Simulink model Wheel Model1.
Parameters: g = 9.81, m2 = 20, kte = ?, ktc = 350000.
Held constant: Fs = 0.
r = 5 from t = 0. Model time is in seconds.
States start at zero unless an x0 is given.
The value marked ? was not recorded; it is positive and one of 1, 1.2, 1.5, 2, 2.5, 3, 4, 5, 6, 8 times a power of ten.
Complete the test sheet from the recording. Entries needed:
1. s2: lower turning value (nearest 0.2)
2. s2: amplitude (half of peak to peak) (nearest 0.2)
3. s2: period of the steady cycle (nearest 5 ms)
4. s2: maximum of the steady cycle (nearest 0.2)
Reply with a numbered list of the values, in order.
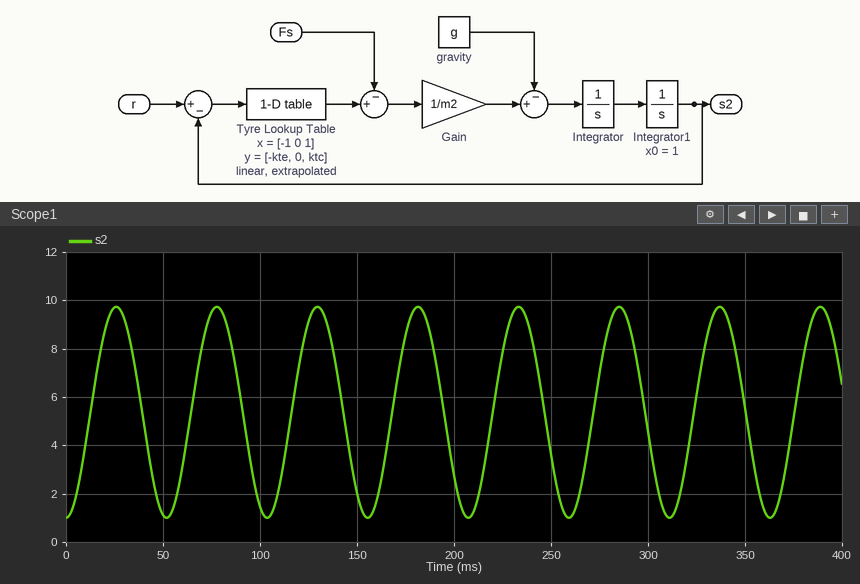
1. 1.0
2. 4.4
3. 50 ms
4. 9.8
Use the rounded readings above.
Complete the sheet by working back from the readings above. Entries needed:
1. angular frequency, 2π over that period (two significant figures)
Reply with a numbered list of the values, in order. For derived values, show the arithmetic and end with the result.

1. 2π / 50 = 0.13 rad/ms
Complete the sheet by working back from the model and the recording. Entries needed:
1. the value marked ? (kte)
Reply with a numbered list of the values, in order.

1. 250000
